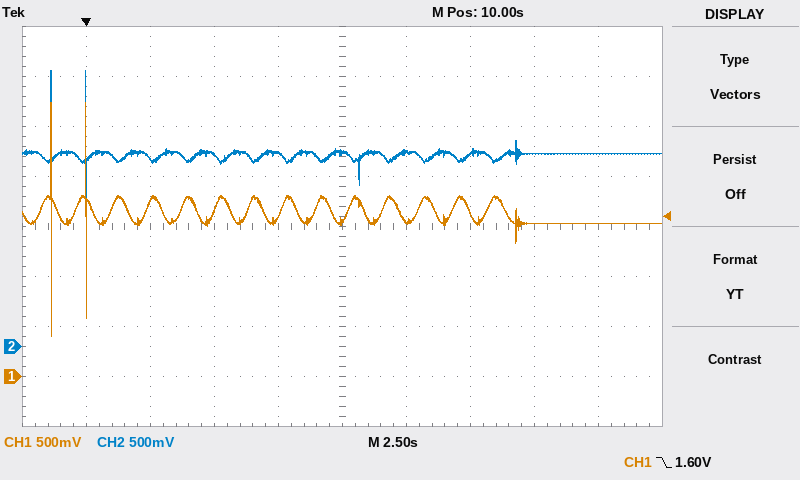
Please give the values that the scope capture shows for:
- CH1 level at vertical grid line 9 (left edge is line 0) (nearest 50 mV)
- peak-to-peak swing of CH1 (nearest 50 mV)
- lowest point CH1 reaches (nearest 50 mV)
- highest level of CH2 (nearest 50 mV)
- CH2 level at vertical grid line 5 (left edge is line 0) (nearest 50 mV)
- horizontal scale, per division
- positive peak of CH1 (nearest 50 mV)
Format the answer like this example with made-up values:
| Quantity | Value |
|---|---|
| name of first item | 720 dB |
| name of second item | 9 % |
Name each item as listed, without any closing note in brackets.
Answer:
| Quantity | Value |
|---|---|
| CH1 level at vertical grid line 9 (left edge is line 0) | 1.55 V |
| peak-to-peak swing of CH1 | 2.35 V |
| lowest point CH1 reaches | 400 mV |
| highest level of CH2 | 2.75 V |
| CH2 level at vertical grid line 5 (left edge is line 0) | 1.95 V |
| horizontal scale, per division | 2.5 s |
| positive peak of CH1 | 2.75 V |
